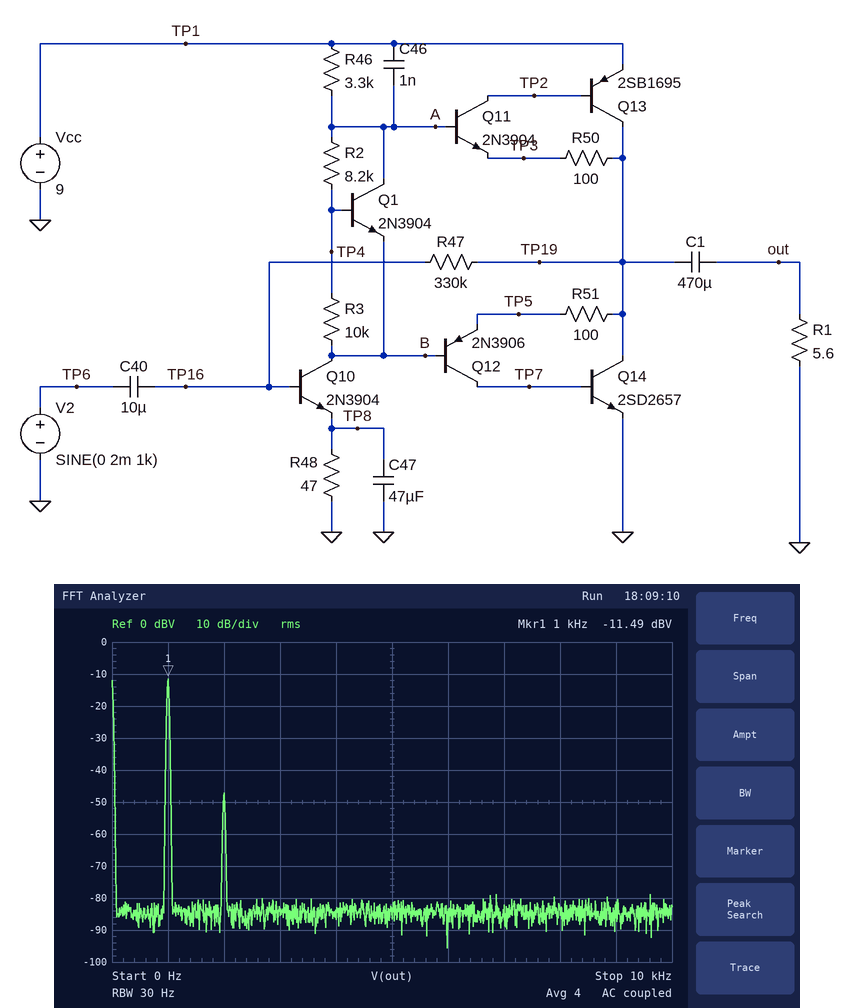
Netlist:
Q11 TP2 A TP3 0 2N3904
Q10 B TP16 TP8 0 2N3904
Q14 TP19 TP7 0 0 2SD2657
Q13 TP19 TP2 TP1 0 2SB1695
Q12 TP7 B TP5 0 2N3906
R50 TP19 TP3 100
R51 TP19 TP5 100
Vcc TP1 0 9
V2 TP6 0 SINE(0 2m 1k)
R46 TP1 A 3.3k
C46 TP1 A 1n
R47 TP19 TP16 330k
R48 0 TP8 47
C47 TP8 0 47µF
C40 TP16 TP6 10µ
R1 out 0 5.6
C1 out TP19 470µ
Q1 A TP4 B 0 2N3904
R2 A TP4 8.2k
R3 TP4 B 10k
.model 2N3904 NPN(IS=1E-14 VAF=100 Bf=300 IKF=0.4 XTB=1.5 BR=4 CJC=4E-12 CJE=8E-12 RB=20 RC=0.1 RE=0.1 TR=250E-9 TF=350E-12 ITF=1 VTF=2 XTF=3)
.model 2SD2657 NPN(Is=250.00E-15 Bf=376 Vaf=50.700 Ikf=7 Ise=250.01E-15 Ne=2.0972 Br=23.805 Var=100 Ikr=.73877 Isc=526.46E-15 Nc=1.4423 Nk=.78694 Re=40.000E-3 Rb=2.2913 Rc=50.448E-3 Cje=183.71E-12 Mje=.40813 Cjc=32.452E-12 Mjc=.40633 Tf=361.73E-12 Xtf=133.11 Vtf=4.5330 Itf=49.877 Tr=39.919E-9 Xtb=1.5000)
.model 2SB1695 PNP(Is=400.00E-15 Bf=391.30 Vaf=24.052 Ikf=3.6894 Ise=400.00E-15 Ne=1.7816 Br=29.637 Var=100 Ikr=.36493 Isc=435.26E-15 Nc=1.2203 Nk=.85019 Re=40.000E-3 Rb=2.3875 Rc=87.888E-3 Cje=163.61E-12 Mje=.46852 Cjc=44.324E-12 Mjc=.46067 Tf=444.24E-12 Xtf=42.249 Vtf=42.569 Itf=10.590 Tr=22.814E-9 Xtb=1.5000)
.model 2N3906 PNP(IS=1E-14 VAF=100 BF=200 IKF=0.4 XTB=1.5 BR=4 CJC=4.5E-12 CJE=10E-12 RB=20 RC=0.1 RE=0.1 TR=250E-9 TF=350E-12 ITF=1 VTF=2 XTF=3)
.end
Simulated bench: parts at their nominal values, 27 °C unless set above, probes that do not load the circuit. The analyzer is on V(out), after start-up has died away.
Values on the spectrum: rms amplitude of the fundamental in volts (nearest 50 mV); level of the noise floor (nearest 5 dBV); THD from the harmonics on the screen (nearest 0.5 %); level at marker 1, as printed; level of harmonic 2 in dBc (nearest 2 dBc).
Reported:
250 mV
-85 dBV
1.5 %
-11.49 dBV
-36 dBc
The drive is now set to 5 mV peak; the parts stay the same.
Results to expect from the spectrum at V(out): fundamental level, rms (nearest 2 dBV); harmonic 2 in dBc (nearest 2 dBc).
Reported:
-4 dBV
-28 dBc
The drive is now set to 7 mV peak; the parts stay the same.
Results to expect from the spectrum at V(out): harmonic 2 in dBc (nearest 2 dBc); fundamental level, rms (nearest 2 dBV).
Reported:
-24 dBc
0 dBV
